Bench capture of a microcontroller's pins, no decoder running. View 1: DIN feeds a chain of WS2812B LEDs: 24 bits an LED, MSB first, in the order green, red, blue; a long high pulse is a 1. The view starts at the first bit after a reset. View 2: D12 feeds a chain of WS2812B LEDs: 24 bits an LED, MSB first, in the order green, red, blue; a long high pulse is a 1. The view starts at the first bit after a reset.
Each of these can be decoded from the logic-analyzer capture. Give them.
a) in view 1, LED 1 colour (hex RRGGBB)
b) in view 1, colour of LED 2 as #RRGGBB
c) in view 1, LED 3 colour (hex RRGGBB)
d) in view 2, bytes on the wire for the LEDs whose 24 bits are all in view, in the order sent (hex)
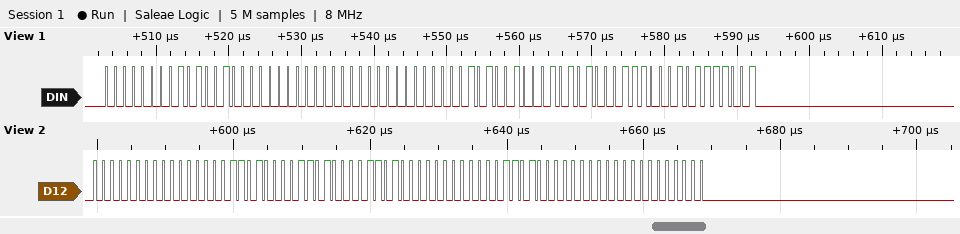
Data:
#A40000
#0000A4
#715479
00 00 D0 D0 D0 00 D0 00 00
